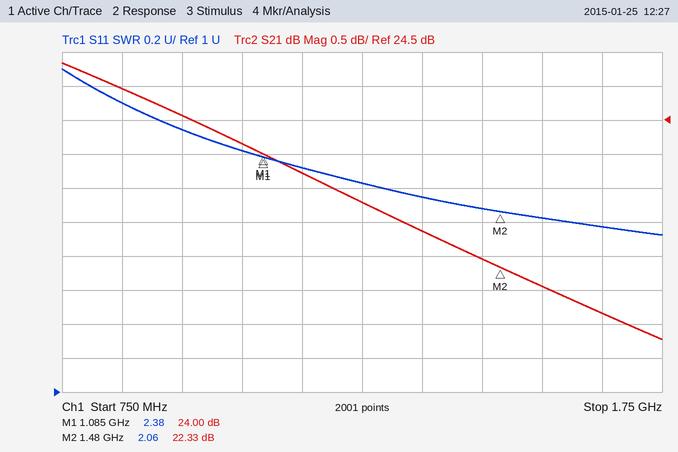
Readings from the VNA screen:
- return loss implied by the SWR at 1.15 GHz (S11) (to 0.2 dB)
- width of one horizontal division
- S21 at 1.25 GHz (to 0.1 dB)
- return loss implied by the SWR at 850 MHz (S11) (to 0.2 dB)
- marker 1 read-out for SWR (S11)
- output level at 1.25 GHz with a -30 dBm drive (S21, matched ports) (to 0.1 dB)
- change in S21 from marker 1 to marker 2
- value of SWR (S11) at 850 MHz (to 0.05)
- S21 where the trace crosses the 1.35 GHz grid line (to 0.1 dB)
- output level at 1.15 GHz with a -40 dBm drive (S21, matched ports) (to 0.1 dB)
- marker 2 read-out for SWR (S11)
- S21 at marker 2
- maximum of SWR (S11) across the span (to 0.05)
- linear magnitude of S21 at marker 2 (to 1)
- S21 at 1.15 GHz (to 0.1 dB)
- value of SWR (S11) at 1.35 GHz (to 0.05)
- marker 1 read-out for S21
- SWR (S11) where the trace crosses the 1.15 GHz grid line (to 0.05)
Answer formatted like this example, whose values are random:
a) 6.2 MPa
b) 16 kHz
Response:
a) 8.0 dB
b) 100 MHz
c) 23.3 dB
d) 6.8 dB
e) 2.38
f) -6.7 dBm
g) -1.67 dB
h) 2.70
i) 22.9 dB
j) -16.3 dBm
k) 2.06
l) 22.33 dB
m) 2.90
n) 13
o) 23.7 dB
p) 2.15
q) 24.00 dB
r) 2.30
